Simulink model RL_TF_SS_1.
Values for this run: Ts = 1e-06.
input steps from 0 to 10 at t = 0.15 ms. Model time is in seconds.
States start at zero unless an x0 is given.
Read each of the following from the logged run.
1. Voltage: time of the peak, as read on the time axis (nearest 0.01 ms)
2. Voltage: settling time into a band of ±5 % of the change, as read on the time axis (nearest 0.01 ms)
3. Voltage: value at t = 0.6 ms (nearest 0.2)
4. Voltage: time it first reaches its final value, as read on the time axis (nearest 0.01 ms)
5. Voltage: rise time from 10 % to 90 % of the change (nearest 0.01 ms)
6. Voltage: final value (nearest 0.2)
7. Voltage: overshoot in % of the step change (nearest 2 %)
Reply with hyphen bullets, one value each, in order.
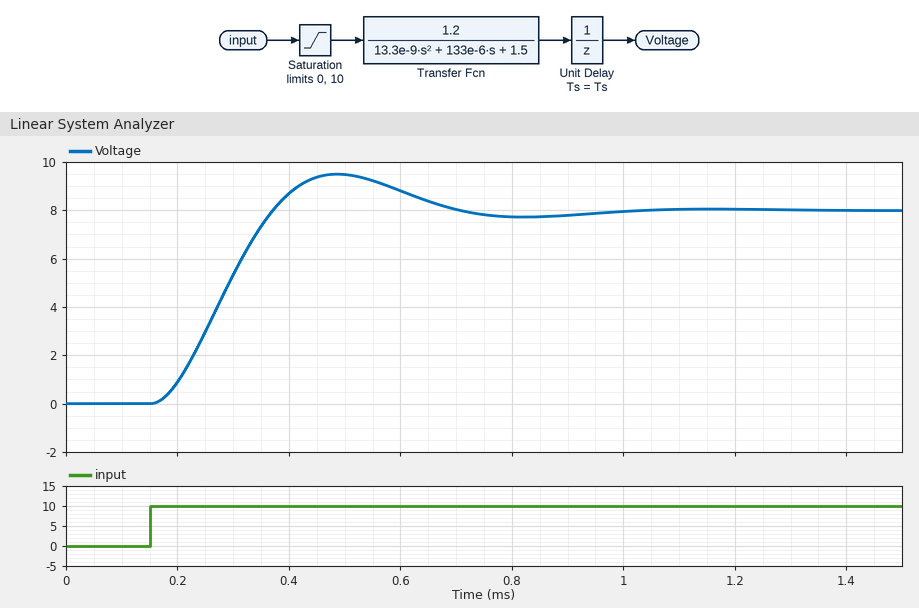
- 0.49 ms
- 0.65 ms
- 8.8
- 0.37 ms
- 0.15 ms
- 8.0
- 18 %
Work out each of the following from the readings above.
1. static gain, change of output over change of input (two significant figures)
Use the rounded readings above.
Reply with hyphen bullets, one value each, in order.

- 0.80
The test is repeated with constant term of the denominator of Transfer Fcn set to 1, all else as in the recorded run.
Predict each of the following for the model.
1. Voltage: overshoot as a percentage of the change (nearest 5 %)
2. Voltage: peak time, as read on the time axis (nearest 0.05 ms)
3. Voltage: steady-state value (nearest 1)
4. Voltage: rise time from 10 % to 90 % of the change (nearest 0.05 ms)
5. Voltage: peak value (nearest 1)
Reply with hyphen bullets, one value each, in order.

- 10 %
- 0.60 ms
- 12
- 0.20 ms
- 13
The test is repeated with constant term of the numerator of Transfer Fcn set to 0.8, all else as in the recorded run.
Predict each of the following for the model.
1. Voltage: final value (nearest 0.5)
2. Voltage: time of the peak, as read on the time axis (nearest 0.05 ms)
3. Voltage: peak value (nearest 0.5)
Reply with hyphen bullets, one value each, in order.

- 5.5
- 0.50 ms
- 6.5
